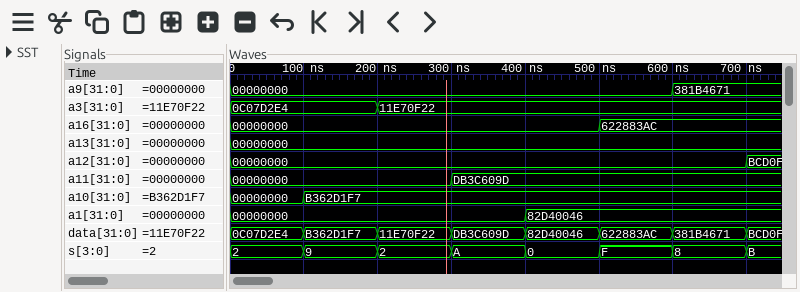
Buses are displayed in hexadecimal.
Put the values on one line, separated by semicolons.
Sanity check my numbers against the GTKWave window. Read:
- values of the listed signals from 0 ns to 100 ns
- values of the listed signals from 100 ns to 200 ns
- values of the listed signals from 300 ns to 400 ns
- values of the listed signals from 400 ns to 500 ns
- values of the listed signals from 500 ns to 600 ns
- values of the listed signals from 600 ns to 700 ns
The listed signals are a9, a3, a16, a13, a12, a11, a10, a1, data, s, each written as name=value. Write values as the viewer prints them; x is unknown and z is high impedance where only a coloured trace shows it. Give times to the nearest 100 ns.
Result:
a9=00000000, a3=0C07D2E4, a16=00000000, a13=00000000, a12=00000000, a11=00000000, a10=00000000, a1=00000000, data=0C07D2E4, s=2; a9=00000000, a3=0C07D2E4, a16=00000000, a13=00000000, a12=00000000, a11=00000000, a10=B362D1F7, a1=00000000, data=B362D1F7, s=9; a9=00000000, a3=11E70F22, a16=00000000, a13=00000000, a12=00000000, a11=DB3C609D, a10=B362D1F7, a1=00000000, data=DB3C609D, s=A; a9=00000000, a3=11E70F22, a16=00000000, a13=00000000, a12=00000000, a11=DB3C609D, a10=B362D1F7, a1=82D40046, data=82D40046, s=0; a9=00000000, a3=11E70F22, a16=622883AC, a13=00000000, a12=00000000, a11=DB3C609D, a10=B362D1F7, a1=82D40046, data=622883AC, s=F; a9=381B4671, a3=11E70F22, a16=622883AC, a13=00000000, a12=00000000, a11=DB3C609D, a10=B362D1F7, a1=82D40046, data=381B4671, s=8
